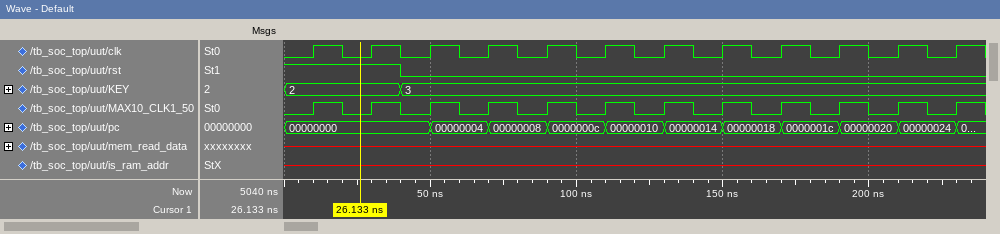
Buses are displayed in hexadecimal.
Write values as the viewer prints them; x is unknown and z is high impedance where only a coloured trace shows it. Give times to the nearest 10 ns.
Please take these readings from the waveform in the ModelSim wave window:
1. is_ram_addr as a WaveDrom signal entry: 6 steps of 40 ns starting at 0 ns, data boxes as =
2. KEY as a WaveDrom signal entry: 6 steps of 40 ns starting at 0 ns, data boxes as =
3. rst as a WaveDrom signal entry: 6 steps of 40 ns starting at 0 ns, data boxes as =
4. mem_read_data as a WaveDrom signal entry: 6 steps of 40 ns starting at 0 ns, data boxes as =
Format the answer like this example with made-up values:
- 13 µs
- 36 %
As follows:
- {name: 'is_ram_addr', wave: 'x.....'}
- {name: 'KEY', wave: '==....', data: '2 3'}
- {name: 'rst', wave: '10....'}
- {name: 'mem_read_data', wave: 'x.....'}
